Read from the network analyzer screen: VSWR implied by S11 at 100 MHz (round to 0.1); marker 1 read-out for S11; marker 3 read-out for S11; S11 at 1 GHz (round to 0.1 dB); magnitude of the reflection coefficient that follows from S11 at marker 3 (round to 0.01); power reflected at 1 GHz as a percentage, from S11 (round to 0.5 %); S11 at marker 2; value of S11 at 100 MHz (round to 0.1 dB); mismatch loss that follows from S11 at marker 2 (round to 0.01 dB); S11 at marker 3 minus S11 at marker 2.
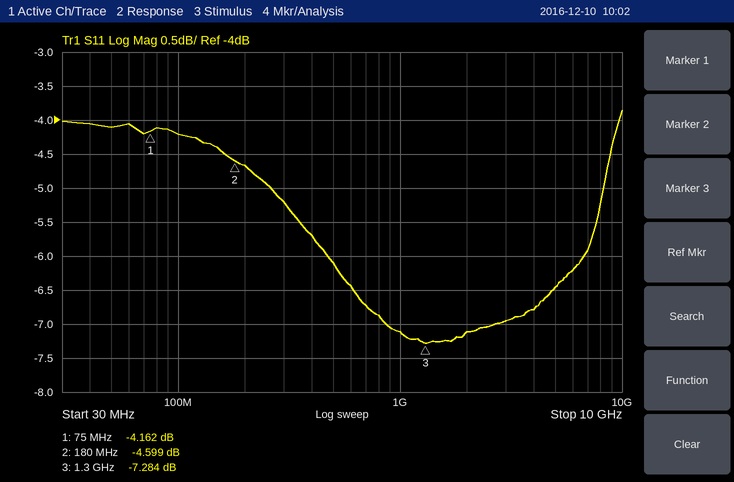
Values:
4.2
-4.162 dB
-7.284 dB
-7.1 dB
0.43
19.5 %
-4.599 dB
-4.2 dB
1.85 dB
-2.685 dB
